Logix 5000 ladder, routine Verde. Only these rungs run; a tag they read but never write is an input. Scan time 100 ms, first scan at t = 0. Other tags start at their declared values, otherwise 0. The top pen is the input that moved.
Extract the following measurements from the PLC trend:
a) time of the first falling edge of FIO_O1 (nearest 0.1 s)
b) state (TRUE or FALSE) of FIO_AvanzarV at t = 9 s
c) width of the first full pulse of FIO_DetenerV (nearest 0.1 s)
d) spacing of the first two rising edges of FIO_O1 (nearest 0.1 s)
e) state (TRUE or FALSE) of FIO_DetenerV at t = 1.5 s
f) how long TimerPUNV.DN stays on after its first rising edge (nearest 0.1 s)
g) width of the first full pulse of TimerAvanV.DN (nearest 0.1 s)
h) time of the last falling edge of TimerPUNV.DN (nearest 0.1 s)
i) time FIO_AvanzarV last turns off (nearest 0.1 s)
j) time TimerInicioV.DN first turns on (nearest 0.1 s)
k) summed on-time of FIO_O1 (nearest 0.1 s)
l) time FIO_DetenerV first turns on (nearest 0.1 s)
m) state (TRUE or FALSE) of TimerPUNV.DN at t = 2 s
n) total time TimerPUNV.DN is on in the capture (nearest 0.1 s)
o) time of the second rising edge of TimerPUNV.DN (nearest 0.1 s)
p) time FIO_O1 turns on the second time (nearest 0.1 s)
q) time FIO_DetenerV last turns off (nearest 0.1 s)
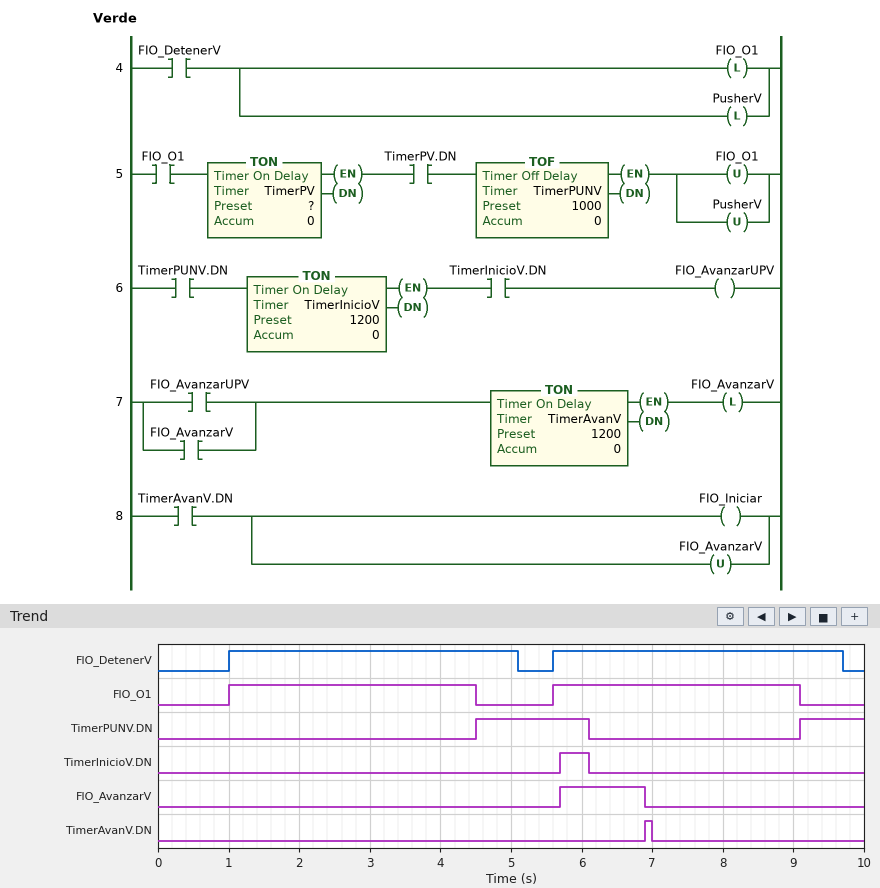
4.5 s
FALSE
4.1 s
4.6 s
TRUE
1.6 s
0.1 s
6.1 s
6.9 s
5.7 s
7.0 s
1.0 s
FALSE
2.5 s
9.1 s
5.6 s
9.7 s
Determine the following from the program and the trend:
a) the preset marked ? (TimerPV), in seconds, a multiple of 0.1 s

3.5 s
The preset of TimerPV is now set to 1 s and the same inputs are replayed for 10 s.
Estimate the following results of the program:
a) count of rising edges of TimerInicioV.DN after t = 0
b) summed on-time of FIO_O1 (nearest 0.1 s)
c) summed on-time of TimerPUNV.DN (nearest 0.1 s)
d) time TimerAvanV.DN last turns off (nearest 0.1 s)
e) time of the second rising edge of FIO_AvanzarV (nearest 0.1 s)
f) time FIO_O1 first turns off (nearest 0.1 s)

2
2.0 s
7.5 s
6.1 s
7.8 s
2.0 s
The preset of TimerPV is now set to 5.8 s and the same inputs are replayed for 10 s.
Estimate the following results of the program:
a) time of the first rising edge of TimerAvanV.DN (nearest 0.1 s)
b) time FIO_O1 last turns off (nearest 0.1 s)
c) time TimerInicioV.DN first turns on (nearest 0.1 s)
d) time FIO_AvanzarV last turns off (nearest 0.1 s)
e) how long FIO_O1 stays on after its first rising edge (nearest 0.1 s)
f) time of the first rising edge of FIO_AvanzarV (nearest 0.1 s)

9.2 s
6.8 s
8.0 s
9.2 s
5.8 s
8.0 s
